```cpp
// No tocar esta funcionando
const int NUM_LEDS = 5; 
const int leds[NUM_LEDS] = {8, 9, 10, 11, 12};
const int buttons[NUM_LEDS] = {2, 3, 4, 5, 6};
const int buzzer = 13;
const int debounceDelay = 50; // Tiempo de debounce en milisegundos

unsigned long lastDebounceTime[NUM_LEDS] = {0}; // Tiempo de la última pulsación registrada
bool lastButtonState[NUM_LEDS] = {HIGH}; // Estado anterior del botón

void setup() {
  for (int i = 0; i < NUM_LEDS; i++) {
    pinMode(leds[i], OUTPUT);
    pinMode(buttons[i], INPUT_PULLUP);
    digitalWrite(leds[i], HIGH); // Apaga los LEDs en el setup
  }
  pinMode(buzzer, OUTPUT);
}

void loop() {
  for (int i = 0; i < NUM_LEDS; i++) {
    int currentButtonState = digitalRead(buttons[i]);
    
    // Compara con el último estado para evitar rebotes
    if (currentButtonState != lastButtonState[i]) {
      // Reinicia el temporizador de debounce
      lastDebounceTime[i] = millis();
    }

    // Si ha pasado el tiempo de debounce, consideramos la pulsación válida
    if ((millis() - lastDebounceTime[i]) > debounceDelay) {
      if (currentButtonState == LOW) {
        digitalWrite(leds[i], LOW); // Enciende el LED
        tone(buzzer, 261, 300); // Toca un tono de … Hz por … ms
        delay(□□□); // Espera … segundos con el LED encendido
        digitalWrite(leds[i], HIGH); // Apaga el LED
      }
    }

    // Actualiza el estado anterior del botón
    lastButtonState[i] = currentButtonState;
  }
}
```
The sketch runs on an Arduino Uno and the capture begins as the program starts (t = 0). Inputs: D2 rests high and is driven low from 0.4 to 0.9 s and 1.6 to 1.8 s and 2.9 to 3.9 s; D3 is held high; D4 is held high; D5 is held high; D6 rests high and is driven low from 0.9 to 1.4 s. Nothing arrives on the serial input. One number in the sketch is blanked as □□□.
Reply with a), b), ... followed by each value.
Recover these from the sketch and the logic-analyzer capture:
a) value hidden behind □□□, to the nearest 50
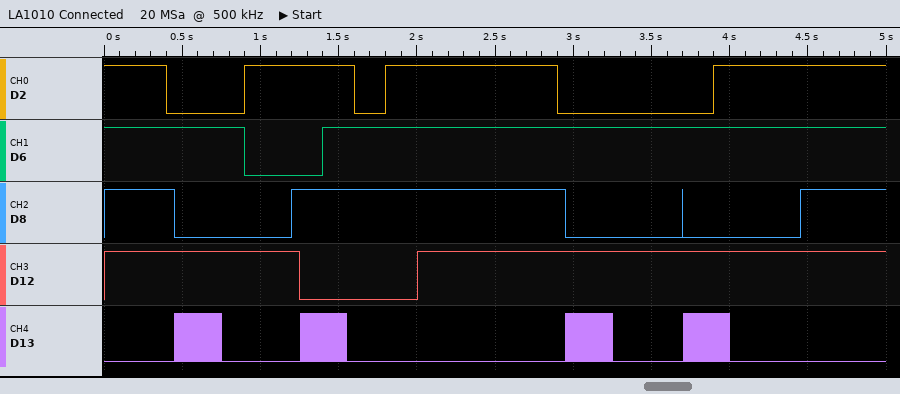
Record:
a) 750
